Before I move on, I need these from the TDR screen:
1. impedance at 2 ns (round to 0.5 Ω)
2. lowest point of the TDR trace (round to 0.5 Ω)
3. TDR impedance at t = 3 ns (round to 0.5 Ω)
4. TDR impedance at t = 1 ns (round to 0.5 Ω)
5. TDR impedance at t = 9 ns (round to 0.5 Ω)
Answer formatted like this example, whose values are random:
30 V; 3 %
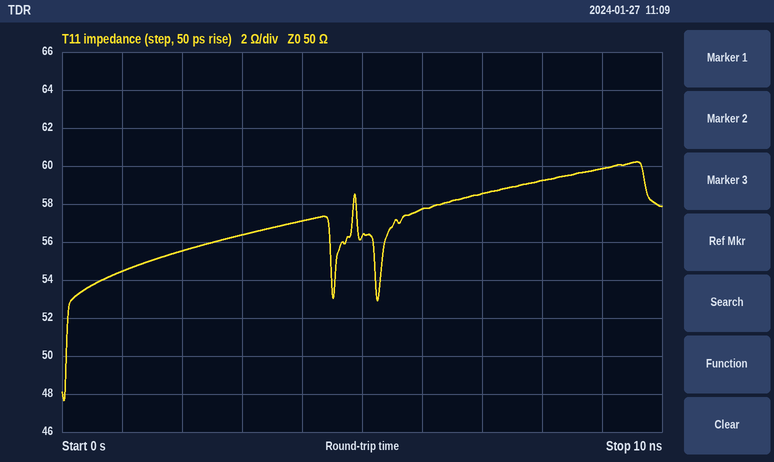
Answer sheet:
55.5 Ω; 47.5 Ω; 56.5 Ω; 54.5 Ω; 60.0 Ω
